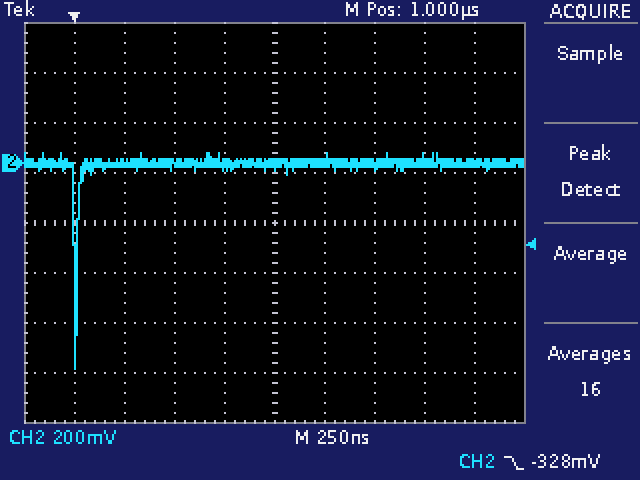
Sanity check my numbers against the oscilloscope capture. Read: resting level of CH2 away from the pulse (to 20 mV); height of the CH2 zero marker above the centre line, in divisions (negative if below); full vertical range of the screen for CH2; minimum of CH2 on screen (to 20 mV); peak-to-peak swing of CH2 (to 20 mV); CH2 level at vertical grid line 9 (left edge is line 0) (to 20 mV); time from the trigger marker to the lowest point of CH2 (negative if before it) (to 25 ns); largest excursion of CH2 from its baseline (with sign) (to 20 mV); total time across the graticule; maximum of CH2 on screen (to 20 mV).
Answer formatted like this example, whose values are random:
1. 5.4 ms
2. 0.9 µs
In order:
1. 0 mV
2. +1.2 div
3. 1.6 V
4. -820 mV
5. 860 mV
6. 0 mV
7. 0 ns
8. -820 mV
9. 2.5 µs
10. 40 mV
